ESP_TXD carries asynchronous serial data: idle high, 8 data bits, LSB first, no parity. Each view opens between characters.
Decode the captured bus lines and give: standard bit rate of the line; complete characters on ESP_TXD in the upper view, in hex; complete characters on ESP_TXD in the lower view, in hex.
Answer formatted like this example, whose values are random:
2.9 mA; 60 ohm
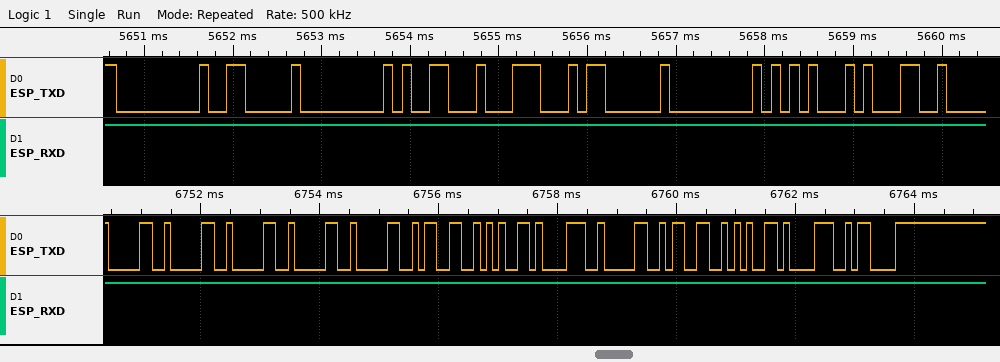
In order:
9600 baud; 00, 06, 00, 19, 1C, 03, 00, 15, 31; 30, 30, 30, 30, 30, 33, 65, 38, 30, 33, 65, 38, C3
